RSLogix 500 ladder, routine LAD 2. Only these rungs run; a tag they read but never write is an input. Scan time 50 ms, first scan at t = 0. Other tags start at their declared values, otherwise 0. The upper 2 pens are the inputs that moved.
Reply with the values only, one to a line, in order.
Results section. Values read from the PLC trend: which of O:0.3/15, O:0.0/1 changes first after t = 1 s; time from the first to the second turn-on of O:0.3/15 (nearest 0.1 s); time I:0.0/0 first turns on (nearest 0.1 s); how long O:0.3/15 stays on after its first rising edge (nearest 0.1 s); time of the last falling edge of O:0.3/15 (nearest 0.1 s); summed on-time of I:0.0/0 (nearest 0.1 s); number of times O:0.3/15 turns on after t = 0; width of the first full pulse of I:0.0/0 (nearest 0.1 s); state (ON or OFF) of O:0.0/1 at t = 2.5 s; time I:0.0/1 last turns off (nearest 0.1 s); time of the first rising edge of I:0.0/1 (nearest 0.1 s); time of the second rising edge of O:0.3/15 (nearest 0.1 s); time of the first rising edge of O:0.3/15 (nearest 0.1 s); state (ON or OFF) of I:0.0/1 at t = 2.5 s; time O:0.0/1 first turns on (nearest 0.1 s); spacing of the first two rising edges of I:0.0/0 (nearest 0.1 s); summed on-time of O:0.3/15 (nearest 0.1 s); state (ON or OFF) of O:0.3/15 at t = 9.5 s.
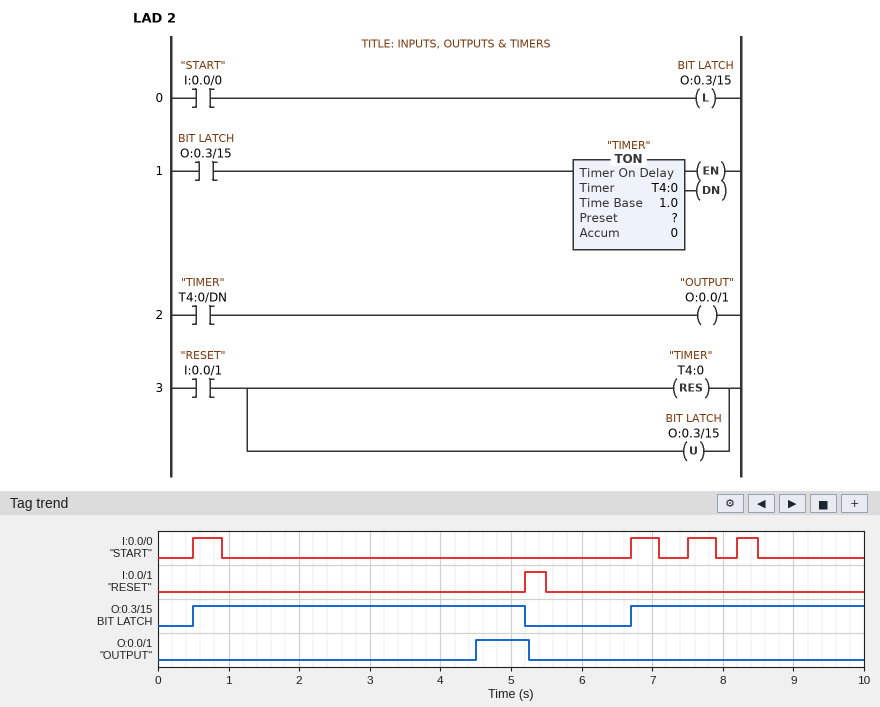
O:0.0/1
6.2 s
0.5 s
4.7 s
5.2 s
1.5 s
2
0.4 s
OFF
5.5 s
5.2 s
6.7 s
0.5 s
OFF
4.5 s
6.2 s
8.0 s
ON
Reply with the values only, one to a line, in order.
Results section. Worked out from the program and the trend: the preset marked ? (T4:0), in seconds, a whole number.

4 s
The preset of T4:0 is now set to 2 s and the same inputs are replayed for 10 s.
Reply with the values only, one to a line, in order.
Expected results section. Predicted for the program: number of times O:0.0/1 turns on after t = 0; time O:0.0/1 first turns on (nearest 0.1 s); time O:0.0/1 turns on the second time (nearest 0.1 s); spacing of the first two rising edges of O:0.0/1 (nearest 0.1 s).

2
2.5 s
8.7 s
6.2 s
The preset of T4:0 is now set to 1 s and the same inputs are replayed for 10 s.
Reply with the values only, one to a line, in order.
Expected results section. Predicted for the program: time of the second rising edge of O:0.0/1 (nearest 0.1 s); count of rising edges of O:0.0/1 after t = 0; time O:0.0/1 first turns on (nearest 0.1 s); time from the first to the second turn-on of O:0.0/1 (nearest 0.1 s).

7.7 s
2
1.5 s
6.2 s
